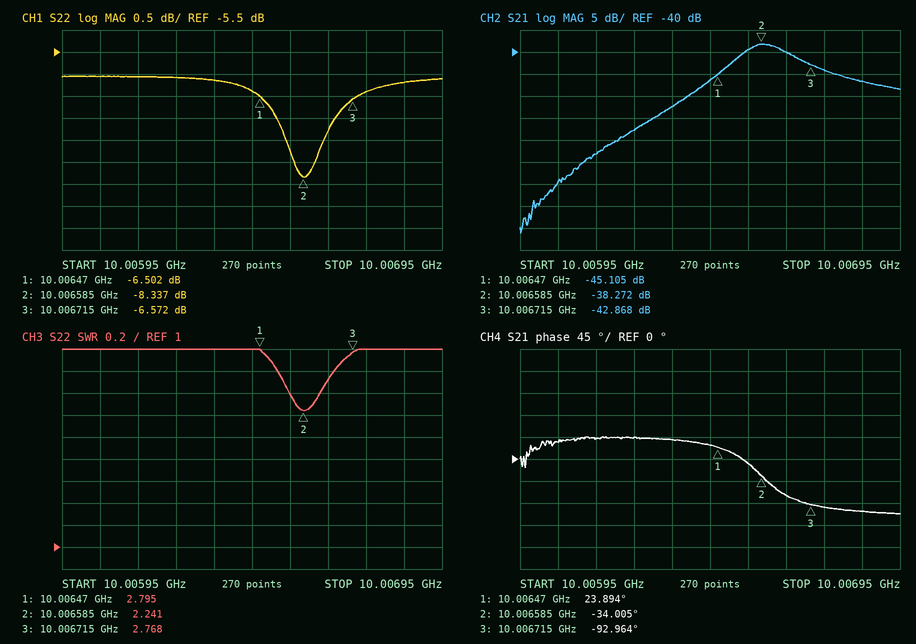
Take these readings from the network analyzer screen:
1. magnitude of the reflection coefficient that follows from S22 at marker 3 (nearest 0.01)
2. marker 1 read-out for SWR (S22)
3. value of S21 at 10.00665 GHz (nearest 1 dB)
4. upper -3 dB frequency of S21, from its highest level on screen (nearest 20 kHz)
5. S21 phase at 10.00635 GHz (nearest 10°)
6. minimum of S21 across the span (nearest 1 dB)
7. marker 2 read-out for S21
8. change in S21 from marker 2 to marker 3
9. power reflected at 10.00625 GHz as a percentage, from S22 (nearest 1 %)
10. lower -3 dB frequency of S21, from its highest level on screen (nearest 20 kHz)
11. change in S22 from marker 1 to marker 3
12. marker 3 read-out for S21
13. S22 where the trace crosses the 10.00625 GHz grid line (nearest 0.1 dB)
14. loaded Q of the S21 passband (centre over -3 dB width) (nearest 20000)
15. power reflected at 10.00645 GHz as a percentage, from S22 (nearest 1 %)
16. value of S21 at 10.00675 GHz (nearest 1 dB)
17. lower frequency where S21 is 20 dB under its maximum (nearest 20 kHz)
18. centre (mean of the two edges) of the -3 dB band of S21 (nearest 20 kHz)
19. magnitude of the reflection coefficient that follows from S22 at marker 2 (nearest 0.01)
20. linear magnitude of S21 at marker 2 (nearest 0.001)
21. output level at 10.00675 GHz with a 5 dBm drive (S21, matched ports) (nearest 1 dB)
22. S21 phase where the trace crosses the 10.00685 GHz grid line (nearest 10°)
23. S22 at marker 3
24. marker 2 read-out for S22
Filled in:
0.47
2.795
-40 dB
10.00668 GHz
40°
-81 dB
-38.272 dB
-4.596 dB
25 %
10.00652 GHz
-0.070 dB
-42.868 dB
-6.1 dB
60000
23 %
-44 dB
10.00624 GHz
10.00660 GHz
0.38
0.012
-39 dBm
-110°
-6.572 dB
-8.337 dB
